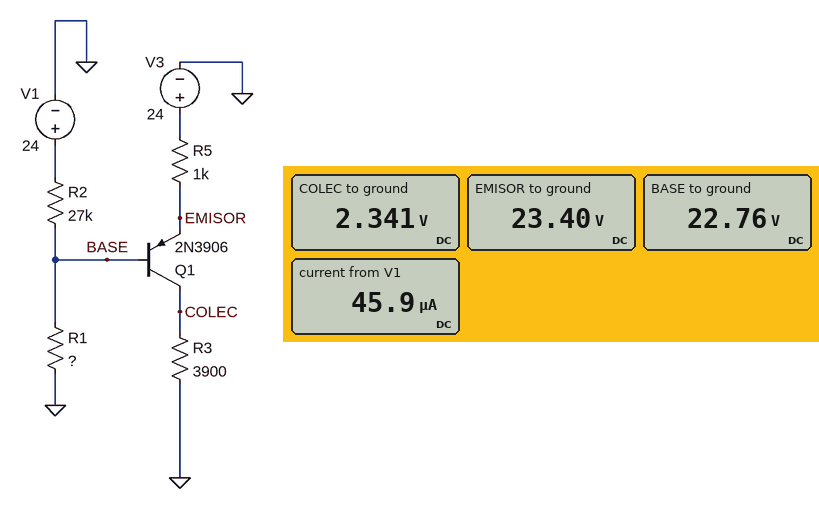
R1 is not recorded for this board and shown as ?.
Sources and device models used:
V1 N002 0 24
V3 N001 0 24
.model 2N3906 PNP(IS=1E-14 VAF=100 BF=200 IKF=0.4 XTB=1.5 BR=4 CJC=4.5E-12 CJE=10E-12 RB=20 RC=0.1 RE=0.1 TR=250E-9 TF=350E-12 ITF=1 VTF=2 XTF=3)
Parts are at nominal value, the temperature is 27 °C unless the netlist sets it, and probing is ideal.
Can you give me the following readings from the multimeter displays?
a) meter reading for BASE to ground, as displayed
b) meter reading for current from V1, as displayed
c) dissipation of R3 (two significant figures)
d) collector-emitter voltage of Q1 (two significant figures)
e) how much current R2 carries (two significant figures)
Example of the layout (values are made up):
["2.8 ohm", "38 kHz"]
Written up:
["22.76 V", "45.9 µA", "1.4 mW", "-21 V", "46 µA"]
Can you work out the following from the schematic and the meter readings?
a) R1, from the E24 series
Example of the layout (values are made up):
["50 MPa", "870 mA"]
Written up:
["470 kΩ"]
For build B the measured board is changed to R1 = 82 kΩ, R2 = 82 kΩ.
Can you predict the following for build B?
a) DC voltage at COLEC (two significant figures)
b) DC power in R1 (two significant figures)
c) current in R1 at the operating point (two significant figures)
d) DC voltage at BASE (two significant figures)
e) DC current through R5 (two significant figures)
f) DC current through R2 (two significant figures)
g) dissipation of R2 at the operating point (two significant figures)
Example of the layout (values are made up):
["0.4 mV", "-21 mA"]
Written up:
["19 V", "4.1 mW", "220 µA", "18 V", "5.0 mA", "70 µA", "400 µW"]
